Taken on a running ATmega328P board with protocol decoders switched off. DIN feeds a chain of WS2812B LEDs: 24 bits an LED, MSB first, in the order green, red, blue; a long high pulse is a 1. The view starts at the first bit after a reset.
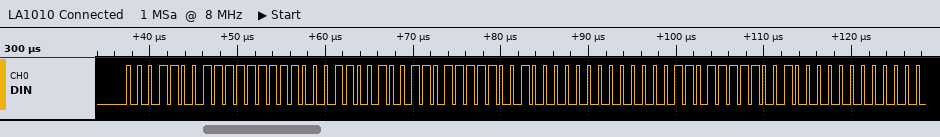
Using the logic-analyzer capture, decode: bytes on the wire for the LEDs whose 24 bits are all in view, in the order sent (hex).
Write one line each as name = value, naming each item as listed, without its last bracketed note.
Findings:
bytes on the wire for the LEDs whose 24 bits are all in view, in the order sent = 19 FF 19 37 C8 00 37 C8 00
